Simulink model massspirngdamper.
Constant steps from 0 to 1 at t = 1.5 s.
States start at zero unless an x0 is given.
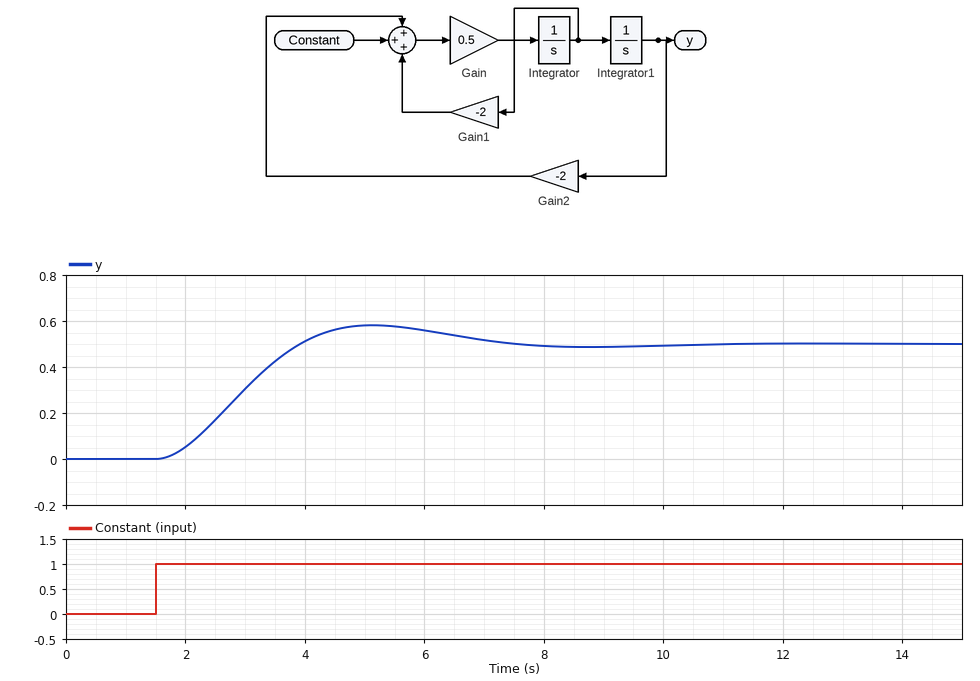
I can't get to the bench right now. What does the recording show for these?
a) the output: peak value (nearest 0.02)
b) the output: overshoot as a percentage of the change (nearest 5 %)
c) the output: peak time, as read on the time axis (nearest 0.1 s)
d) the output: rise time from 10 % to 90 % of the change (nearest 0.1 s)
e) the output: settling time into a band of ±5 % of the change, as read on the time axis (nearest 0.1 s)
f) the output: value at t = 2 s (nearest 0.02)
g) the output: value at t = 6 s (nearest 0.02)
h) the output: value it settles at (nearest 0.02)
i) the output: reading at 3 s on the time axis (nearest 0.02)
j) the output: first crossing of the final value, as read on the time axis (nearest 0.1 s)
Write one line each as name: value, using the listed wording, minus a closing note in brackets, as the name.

the output: peak value: 0.58
the output: overshoot as a percentage of the change: 15 %
the output: peak time, as read on the time axis: 5.1 s
the output: rise time from 10 % to 90 % of the change: 1.6 s
the output: settling time into a band of ±5 % of the change, as read on the time axis: 6.8 s
the output: value at t = 2 s: 0.06
the output: value at t = 6 s: 0.56
the output: value it settles at: 0.50
the output: reading at 3 s on the time axis: 0.30
the output: first crossing of the final value, as read on the time axis: 3.9 s
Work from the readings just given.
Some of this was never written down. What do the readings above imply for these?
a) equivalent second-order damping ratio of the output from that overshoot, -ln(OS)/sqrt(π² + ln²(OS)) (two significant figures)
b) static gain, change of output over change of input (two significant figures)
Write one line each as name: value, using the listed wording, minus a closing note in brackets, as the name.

equivalent second-order damping ratio of the output from that overshoot, -ln(OS)/sqrt(π² + ln²(OS)): 0.52
static gain, change of output over change of input: 0.50
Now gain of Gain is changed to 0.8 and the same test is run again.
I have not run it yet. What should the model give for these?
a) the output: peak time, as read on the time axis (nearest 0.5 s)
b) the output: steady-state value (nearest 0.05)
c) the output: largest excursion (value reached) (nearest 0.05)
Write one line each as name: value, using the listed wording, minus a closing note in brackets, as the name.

the output: peak time, as read on the time axis: 4.5 s
the output: steady-state value: 0.50
the output: largest excursion (value reached): 0.55
